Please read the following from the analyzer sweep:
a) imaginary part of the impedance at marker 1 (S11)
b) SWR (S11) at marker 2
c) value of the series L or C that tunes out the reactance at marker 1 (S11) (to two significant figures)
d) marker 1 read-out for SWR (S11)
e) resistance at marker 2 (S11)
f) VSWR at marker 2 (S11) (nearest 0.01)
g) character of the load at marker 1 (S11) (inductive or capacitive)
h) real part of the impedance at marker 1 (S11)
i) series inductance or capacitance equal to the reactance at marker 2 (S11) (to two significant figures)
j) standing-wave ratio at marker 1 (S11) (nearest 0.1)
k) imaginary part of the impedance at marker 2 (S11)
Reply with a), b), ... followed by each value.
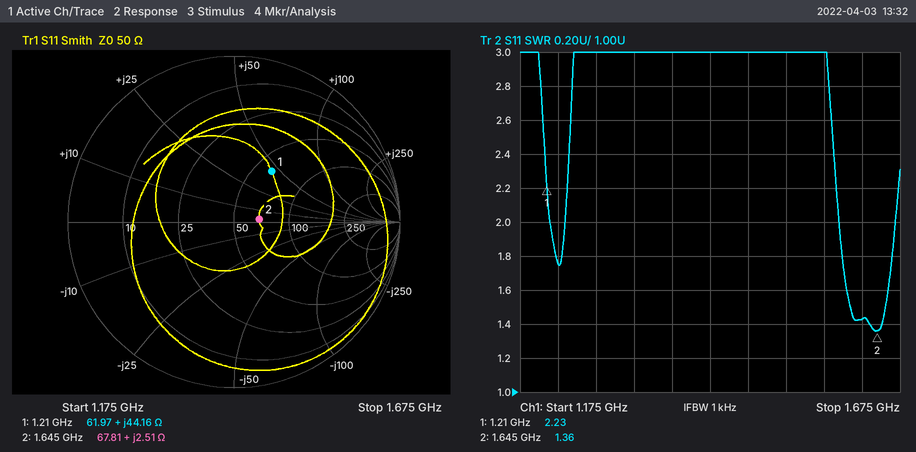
a) +44.16 Ω
b) 1.36
c) 3.0 pF
d) 2.23
e) 67.81 Ω
f) 1.36
g) inductive
h) 61.97 Ω
i) 240 pH
j) 2.2
k) +2.51 Ω
